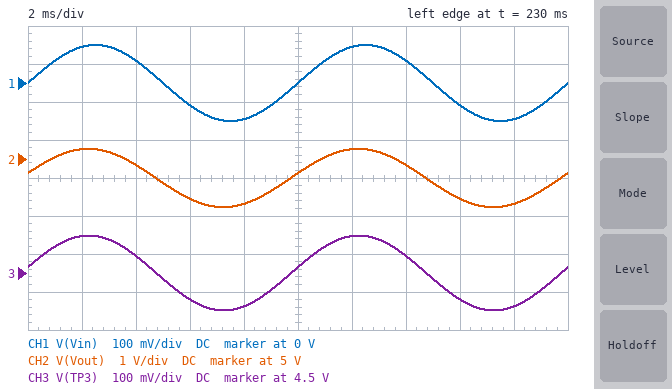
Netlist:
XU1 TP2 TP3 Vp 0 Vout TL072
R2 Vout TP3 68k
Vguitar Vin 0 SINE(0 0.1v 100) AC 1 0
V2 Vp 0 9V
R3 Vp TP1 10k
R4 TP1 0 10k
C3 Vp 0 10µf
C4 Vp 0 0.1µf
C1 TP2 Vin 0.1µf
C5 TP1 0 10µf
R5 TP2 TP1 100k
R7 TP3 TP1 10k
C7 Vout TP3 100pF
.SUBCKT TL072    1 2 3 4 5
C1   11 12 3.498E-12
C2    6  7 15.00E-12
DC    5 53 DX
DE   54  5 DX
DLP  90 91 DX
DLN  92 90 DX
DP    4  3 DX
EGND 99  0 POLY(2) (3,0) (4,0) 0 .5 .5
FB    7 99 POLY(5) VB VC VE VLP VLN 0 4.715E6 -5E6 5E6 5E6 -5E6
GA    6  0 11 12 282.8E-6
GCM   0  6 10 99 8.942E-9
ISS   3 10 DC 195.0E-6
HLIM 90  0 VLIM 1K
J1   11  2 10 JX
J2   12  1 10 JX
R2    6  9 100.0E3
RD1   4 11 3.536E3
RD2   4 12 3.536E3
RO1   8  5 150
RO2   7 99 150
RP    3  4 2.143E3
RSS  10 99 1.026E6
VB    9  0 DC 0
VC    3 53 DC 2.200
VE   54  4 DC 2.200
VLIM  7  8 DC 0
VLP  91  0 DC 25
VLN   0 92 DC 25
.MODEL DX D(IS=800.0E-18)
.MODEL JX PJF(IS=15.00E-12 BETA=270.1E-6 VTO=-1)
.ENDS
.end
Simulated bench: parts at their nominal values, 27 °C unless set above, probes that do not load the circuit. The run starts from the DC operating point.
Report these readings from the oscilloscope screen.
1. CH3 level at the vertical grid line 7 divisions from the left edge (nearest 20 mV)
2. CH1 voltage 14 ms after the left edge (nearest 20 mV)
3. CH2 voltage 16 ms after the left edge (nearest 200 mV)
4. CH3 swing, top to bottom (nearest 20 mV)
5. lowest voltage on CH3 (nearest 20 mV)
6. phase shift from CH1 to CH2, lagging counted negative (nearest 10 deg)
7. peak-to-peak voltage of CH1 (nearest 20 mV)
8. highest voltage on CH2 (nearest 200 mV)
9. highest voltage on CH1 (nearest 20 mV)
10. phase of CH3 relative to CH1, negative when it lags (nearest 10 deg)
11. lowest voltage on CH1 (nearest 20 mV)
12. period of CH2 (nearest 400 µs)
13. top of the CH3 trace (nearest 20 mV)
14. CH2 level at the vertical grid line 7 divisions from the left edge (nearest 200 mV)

4.54 V
60 mV
4.0 V
200 mV
4.40 V
10 deg
200 mV
5.2 V
100 mV
10 deg
-100 mV
10.0 ms
4.60 V
4.8 V
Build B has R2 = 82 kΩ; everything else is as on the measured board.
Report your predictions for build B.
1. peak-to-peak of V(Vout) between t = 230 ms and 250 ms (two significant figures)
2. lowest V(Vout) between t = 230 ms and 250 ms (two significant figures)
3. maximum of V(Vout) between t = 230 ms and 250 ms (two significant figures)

1.8 V
3.6 V
5.4 V
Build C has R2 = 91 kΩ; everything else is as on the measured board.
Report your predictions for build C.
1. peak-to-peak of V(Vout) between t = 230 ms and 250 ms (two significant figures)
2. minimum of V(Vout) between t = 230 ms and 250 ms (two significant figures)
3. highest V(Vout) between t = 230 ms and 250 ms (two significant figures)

2.0 V
3.5 V
5.5 V
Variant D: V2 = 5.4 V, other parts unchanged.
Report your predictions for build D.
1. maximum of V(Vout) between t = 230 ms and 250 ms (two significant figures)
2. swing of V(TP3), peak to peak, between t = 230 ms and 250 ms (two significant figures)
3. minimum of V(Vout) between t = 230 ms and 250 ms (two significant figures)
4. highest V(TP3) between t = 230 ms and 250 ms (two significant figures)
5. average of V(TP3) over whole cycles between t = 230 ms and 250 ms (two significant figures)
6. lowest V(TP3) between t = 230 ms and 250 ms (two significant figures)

3.5 V
200 mV
1.9 V
2.8 V
2.7 V
2.6 V
